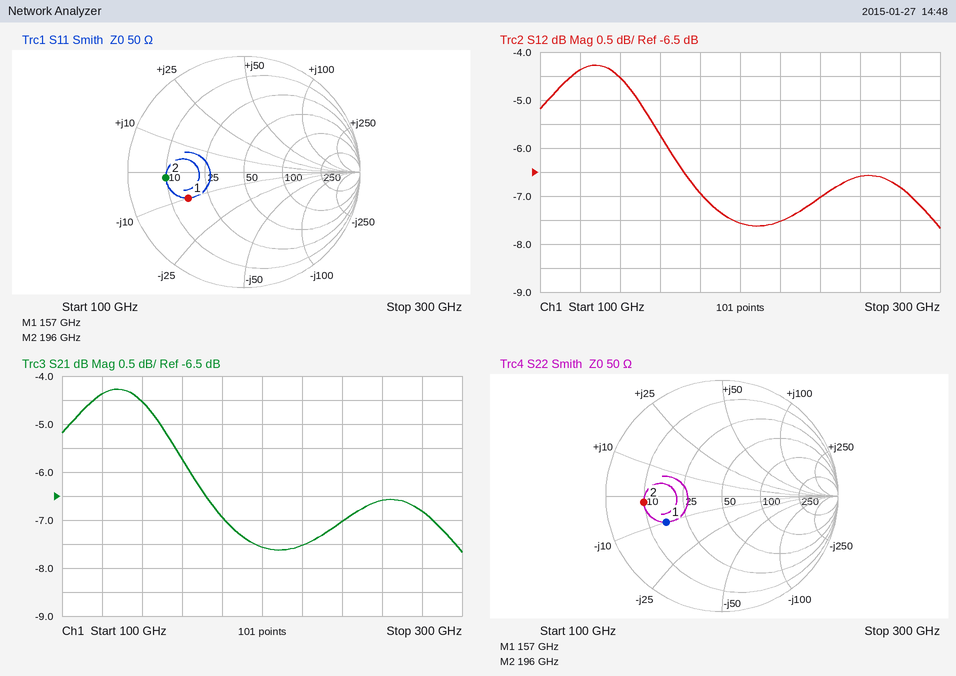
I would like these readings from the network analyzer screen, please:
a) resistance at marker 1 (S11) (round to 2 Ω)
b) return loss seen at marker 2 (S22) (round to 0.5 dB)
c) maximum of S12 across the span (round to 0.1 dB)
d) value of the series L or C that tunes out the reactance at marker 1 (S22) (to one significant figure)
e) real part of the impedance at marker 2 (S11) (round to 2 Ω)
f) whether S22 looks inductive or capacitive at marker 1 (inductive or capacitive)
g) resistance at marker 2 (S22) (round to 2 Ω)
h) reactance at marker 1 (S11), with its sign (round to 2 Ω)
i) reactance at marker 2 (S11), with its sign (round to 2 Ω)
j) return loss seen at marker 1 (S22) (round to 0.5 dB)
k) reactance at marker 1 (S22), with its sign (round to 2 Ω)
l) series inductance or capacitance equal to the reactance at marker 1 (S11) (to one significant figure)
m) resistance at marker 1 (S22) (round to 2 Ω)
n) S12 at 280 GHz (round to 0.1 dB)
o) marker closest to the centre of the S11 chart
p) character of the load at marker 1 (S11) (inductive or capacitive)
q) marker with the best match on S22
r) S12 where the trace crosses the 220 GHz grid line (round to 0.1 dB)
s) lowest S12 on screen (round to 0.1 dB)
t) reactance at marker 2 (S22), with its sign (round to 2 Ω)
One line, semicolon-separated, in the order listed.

16 Ω; 3.5 dB; -4.3 dB; 10 pH; 10 Ω; capacitive; 10 Ω; -10 Ω; -2 Ω; 5.5 dB; -10 Ω; 100 fF; 16 Ω; -6.8 dB; marker 1; capacitive; marker 1; -7.5 dB; -7.7 dB; -2 Ω
